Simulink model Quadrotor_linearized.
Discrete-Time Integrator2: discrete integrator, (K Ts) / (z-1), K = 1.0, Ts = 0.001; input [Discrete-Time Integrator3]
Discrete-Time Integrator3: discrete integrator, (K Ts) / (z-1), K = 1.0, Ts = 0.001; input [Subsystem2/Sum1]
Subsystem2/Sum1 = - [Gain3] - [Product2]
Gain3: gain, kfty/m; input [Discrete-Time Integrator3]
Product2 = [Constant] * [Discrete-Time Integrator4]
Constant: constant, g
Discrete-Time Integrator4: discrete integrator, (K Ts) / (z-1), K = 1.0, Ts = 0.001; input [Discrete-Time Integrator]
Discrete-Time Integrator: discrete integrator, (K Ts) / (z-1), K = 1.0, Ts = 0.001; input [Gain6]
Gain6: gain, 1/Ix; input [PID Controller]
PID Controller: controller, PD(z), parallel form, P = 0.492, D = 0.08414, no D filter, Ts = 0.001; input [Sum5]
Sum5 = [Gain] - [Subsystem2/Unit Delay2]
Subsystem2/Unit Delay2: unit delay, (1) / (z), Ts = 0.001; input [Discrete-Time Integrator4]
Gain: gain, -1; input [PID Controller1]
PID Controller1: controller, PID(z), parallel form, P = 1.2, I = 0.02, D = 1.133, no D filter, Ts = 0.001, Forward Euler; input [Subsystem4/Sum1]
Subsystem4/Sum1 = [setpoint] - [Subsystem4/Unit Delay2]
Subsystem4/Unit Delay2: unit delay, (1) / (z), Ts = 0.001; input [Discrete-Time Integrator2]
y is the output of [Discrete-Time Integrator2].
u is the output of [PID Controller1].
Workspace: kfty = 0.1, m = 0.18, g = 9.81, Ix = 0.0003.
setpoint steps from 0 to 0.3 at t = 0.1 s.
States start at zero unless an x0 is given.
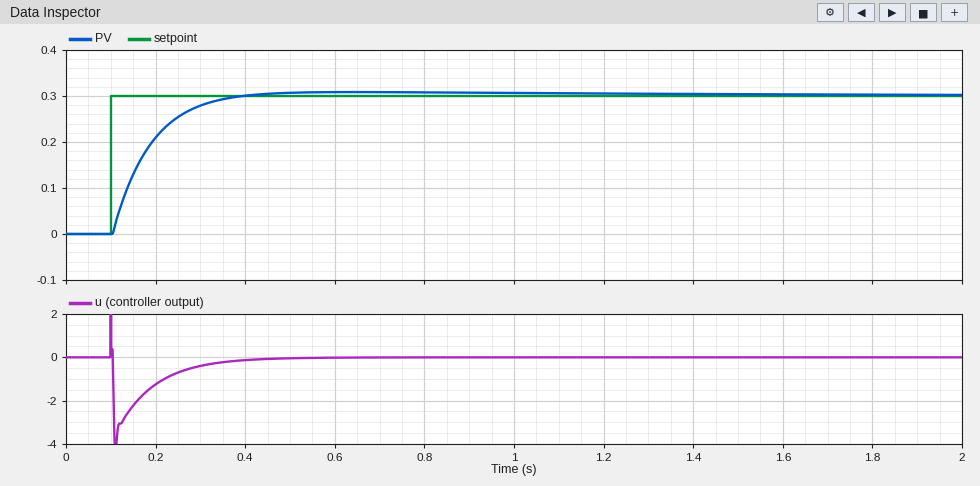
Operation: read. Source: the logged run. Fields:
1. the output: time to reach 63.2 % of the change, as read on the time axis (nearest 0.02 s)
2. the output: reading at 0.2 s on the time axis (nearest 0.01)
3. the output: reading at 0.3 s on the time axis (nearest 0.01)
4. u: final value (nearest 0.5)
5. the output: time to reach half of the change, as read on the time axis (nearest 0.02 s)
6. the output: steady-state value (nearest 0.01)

0.18 s
0.21
0.28
0.0
0.16 s
0.30
